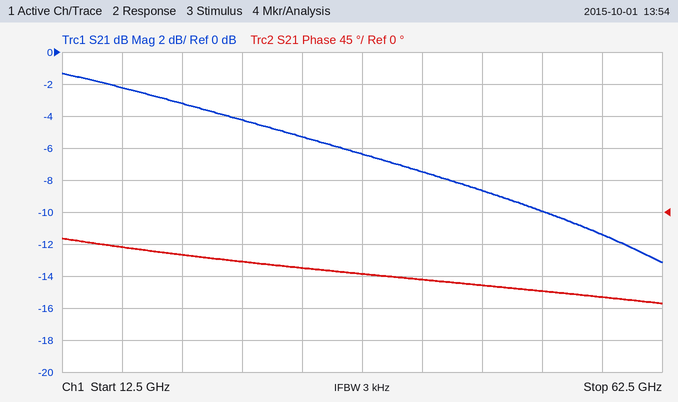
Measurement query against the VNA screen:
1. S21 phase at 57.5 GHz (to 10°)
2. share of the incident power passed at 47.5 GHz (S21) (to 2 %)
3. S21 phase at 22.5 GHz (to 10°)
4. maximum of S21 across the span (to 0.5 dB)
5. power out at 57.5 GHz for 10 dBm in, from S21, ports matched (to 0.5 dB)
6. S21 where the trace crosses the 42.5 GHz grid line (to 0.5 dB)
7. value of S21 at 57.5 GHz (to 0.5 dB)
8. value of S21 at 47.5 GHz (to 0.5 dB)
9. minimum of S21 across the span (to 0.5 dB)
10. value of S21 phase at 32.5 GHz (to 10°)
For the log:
-120°
14 %
-60°
-1.5 dB
-1.5 dBm
-7.5 dB
-11.5 dB
-8.5 dB
-13.0 dB
-80°
